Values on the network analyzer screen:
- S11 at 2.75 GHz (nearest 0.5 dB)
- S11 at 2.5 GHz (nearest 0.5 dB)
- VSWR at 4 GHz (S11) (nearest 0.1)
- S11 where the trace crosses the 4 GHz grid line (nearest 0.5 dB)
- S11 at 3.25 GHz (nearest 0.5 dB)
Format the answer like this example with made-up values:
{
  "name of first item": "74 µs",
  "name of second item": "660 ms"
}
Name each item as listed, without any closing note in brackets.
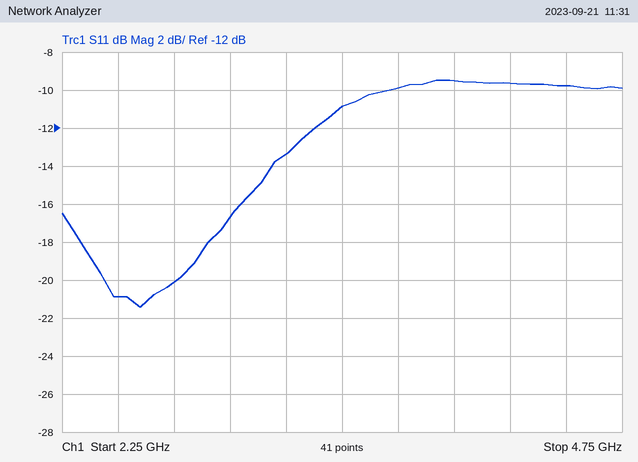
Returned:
{
  "S11 at 2.75 GHz": "-20.0 dB",
  "S11 at 2.5 GHz": "-21.0 dB",
  "VSWR at 4 GHz (S11)": "2.0",
  "S11 where the trace crosses the 4 GHz grid line": "-9.5 dB",
  "S11 at 3.25 GHz": "-13.5 dB"
}
